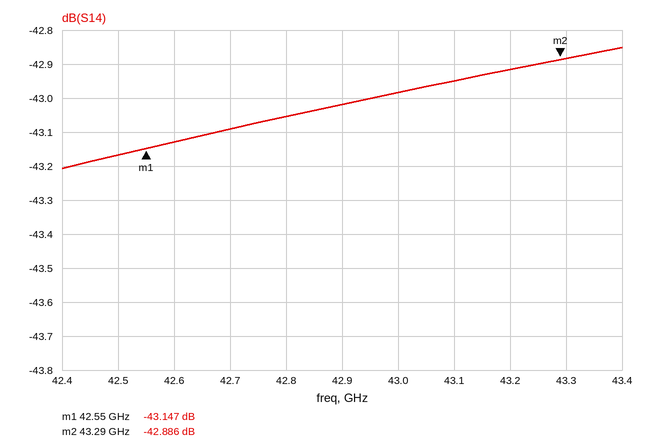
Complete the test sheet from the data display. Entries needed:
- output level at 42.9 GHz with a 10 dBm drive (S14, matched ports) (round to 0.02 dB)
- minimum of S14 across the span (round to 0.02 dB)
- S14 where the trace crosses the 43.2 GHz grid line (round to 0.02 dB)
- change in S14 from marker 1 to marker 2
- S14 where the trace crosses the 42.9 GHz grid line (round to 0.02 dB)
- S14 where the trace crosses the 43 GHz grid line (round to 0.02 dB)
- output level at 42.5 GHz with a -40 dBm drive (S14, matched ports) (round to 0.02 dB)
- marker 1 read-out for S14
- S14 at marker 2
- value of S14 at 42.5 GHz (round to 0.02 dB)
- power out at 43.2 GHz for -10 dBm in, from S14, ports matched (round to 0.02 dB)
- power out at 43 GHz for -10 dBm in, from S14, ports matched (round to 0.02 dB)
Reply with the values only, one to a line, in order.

-33.02 dBm
-43.20 dB
-42.92 dB
0.261 dB
-43.02 dB
-42.98 dB
-83.16 dBm
-43.147 dB
-42.886 dB
-43.16 dB
-52.92 dBm
-52.98 dBm
